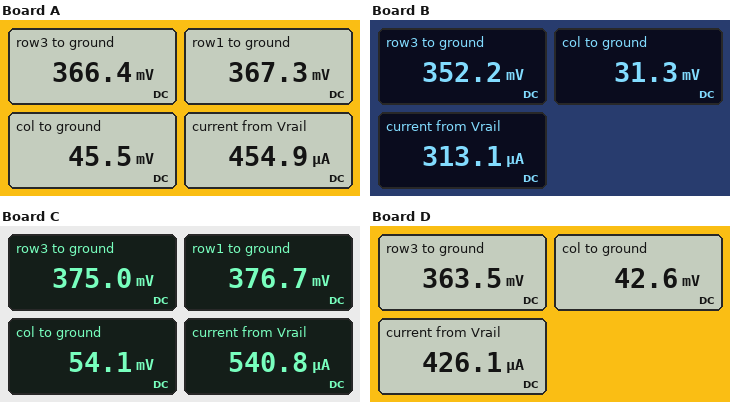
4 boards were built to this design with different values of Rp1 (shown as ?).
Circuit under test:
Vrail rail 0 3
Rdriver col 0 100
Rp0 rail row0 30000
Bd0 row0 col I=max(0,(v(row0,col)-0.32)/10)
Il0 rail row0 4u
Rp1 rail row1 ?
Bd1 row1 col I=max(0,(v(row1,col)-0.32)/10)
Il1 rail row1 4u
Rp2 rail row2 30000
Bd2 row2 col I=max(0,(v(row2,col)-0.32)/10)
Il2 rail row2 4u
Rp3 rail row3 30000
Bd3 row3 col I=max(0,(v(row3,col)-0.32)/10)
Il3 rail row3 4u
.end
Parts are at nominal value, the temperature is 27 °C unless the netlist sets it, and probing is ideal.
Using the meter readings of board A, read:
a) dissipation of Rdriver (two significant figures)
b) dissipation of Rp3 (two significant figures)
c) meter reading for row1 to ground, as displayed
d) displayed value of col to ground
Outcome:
21 µW
230 µW
367.3 mV
45.5 mV
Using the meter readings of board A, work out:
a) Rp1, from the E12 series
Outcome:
15 kΩ
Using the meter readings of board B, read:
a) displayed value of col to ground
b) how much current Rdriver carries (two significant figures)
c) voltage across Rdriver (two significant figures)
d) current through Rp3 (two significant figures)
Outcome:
31.3 mV
310 µA
31 mV
88 µA
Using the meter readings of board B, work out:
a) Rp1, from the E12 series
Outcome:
82 kΩ
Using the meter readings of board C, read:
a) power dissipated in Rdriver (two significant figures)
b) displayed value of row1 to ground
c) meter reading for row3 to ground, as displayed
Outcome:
29 µW
376.7 mV
375.0 mV
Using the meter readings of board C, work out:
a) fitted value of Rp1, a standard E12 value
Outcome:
10 kΩ
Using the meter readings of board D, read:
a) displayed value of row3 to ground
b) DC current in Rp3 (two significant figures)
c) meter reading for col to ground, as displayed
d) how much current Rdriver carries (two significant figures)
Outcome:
363.5 mV
88 µA
42.6 mV
430 µA
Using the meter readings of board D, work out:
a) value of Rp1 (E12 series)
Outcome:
18 kΩ
